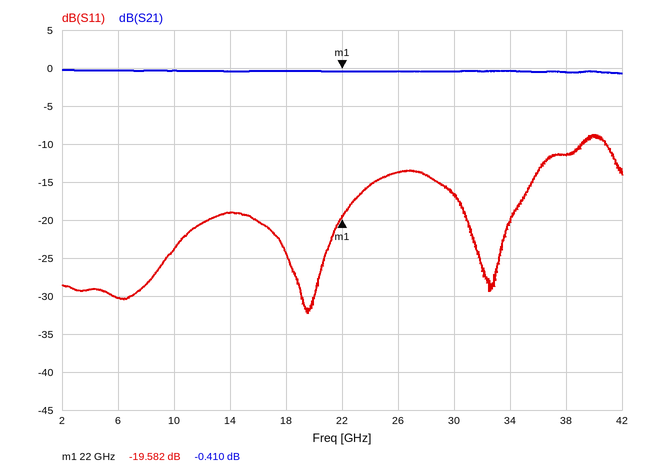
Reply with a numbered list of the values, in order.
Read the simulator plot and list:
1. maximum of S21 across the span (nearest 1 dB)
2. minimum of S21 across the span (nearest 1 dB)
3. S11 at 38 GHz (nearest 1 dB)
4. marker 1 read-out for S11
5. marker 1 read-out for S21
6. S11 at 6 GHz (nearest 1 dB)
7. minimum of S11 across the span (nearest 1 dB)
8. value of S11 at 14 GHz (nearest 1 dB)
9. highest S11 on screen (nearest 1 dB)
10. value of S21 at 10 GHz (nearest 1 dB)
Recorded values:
1. 0 dB
2. -1 dB
3. -11 dB
4. -19.582 dB
5. -0.410 dB
6. -30 dB
7. -32 dB
8. -19 dB
9. -9 dB
10. 0 dB
